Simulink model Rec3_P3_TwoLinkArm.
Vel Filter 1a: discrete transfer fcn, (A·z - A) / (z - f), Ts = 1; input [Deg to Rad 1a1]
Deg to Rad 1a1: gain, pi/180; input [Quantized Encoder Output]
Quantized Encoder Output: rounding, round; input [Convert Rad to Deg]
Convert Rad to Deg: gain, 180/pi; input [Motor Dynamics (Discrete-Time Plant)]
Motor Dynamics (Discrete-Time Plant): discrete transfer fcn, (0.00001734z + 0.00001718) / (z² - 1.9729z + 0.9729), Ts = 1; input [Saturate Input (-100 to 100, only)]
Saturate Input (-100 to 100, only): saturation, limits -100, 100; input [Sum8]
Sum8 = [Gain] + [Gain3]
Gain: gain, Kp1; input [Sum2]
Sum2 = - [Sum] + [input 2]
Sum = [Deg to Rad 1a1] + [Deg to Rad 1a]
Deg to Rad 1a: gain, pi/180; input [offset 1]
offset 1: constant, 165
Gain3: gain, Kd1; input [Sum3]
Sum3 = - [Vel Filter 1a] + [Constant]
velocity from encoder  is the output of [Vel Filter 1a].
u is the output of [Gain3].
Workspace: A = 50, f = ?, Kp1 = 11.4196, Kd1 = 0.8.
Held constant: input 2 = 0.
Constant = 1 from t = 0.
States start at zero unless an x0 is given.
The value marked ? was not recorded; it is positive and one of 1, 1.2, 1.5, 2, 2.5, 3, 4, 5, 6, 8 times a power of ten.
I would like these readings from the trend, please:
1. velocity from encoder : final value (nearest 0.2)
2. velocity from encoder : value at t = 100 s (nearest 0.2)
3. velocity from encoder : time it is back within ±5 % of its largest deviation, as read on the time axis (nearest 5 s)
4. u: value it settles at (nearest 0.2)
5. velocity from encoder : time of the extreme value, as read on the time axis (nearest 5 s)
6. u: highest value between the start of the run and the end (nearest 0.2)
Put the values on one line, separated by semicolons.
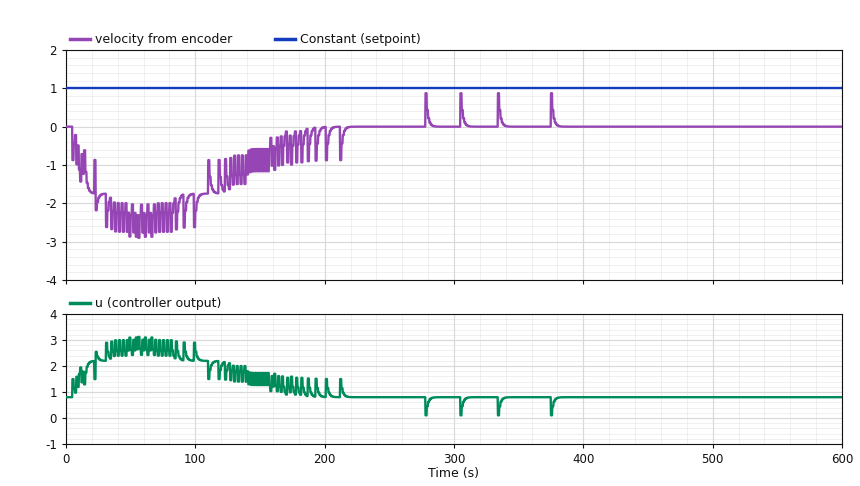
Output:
0.0; -2.2; 380 s; 0.8; 55 s; 3.2
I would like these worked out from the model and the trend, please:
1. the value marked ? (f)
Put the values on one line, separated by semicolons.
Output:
0.5
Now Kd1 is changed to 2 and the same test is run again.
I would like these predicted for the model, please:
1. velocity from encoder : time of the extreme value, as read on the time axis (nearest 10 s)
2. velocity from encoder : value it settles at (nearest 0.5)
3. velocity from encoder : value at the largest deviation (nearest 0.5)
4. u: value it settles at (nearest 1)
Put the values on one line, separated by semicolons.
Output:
70 s; 0.0; -2.5; 2
